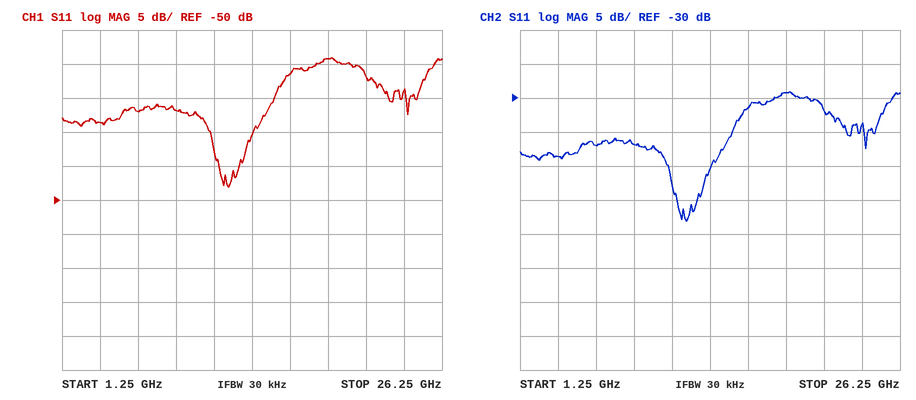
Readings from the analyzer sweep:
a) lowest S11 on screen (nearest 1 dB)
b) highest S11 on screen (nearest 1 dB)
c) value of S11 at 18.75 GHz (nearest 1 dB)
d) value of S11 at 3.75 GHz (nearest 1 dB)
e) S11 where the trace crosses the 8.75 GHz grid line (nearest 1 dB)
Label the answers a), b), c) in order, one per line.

a) -48 dB
b) -29 dB
c) -29 dB
d) -39 dB
e) -37 dB
